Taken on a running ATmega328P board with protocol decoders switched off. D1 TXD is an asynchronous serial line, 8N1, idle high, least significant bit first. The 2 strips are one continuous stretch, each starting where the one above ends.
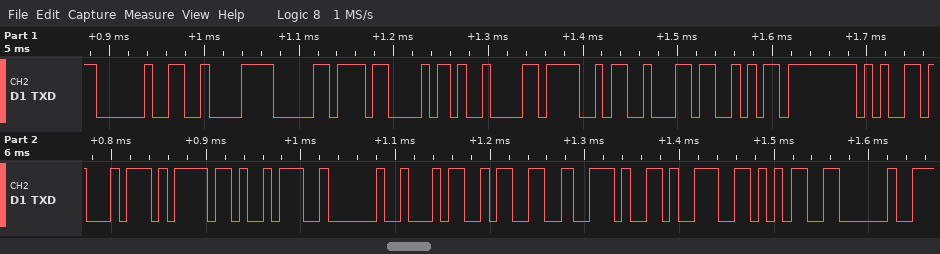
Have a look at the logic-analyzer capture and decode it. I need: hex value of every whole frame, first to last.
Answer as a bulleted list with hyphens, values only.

- 20 C2 B0 43 09 4F 62 6A 65 74 6F 3A 20 34 33 2E 39 35 20
